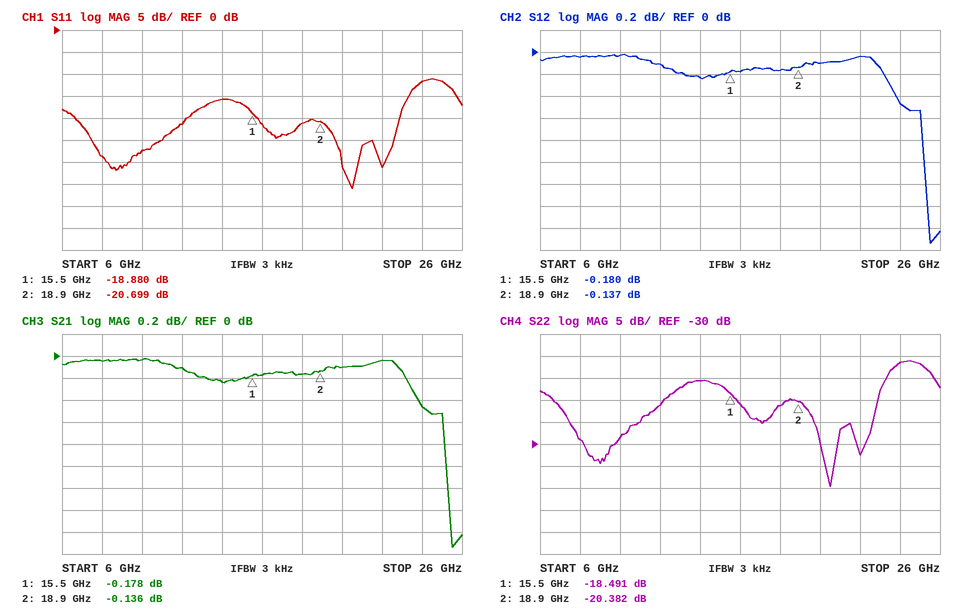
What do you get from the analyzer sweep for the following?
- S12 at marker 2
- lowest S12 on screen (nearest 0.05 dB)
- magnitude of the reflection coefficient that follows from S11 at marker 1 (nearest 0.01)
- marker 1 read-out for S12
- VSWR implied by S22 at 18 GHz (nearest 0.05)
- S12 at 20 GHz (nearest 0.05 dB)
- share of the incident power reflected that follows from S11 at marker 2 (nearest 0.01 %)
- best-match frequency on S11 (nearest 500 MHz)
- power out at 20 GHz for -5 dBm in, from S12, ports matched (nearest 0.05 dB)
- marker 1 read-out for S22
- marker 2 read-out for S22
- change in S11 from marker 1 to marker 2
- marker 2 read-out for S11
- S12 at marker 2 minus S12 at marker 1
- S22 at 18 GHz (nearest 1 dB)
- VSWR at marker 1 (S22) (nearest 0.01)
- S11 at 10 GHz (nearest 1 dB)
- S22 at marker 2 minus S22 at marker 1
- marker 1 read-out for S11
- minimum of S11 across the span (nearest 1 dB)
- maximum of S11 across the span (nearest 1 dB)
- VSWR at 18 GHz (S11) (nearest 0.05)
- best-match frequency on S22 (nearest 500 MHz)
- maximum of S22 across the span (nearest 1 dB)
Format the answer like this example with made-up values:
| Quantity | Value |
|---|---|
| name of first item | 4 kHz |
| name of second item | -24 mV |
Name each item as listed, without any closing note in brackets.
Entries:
| Quantity | Value |
|---|---|
| S12 at marker 2 | -0.137 dB |
| lowest S12 on screen | -1.75 dB |
| magnitude of the reflection coefficient that follows from S11 at marker 1 | 0.11 |
| marker 1 read-out for S12 | -0.180 dB |
| VSWR implied by S22 at 18 GHz | 1.20 |
| S12 at 20 GHz | -0.10 dB |
| share of the incident power reflected that follows from S11 at marker 2 | 0.85 % |
| best-match frequency on S11 | 20.5 GHz |
| power out at 20 GHz for -5 dBm in, from S12, ports matched | -5.10 dBm |
| marker 1 read-out for S22 | -18.491 dB |
| marker 2 read-out for S22 | -20.382 dB |
| change in S11 from marker 1 to marker 2 | -1.819 dB |
| marker 2 read-out for S11 | -20.699 dB |
| S12 at marker 2 minus S12 at marker 1 | 0.043 dB |
| S22 at 18 GHz | -21 dB |
| VSWR at marker 1 (S22) | 1.27 |
| S11 at 10 GHz | -27 dB |
| S22 at marker 2 minus S22 at marker 1 | -1.891 dB |
| marker 1 read-out for S11 | -18.880 dB |
| minimum of S11 across the span | -36 dB |
| maximum of S11 across the span | -11 dB |
| VSWR at 18 GHz (S11) | 1.20 |
| best-match frequency on S22 | 20.5 GHz |
| maximum of S22 across the span | -11 dB |
